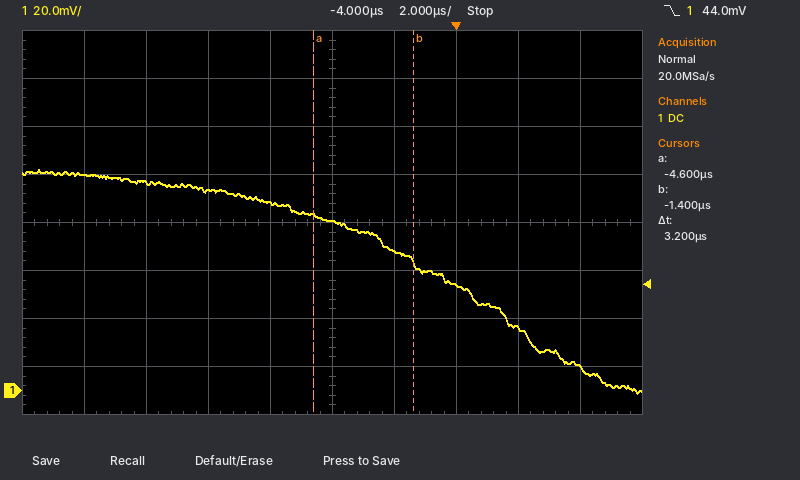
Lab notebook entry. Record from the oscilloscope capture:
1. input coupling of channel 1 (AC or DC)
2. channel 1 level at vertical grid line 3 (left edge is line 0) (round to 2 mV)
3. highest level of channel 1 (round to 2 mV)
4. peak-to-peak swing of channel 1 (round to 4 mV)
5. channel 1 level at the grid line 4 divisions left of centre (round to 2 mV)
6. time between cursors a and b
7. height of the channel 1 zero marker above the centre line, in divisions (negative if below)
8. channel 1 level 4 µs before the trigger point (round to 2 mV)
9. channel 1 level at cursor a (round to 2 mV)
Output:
DC
84 mV
92 mV
92 mV
90 mV
3.2 µs
-3.5 div
70 mV
74 mV
